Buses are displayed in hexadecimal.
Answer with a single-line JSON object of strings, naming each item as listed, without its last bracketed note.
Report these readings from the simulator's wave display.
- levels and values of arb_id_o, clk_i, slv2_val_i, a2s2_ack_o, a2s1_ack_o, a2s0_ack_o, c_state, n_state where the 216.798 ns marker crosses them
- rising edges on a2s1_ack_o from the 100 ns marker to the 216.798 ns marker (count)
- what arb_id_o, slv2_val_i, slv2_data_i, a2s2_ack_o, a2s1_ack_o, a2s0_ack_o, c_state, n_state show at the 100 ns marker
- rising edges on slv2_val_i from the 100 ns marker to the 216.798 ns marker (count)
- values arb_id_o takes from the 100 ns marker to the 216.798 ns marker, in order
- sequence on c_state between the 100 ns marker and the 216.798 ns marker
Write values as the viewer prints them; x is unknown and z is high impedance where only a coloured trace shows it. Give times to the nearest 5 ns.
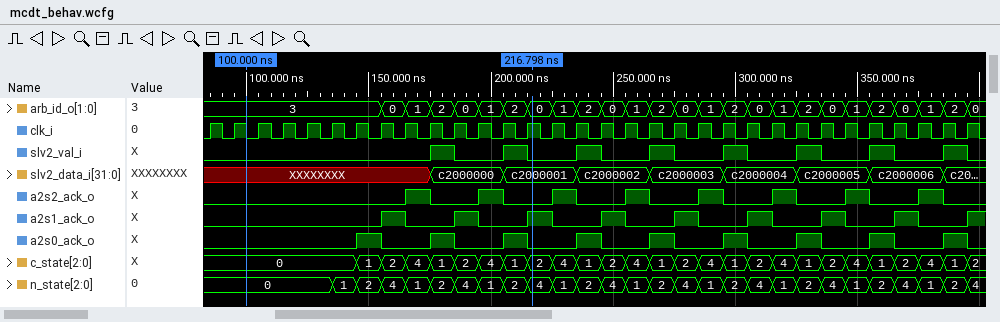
{"levels and values of arb_id_o, clk_i, slv2_val_i, a2s2_ack_o, a2s1_ack_o, a2s0_ack_o, c_state, n_state where the 216.798 ns marker crosses them": "arb_id_o=0, clk_i=1, slv2_val_i=0, a2s2_ack_o=0, a2s1_ack_o=1, a2s0_ack_o=0, c_state=2, n_state=4", "rising edges on a2s1_ack_o from the 100 ns marker to the 216.798 ns marker": "3", "what arb_id_o, slv2_val_i, slv2_data_i, a2s2_ack_o, a2s1_ack_o, a2s0_ack_o, c_state, n_state show at the 100 ns marker": "arb_id_o=3, slv2_val_i=0, slv2_data_i=XXXXXXXX, a2s2_ack_o=0, a2s1_ack_o=0, a2s0_ack_o=0, c_state=0, n_state=0", "rising edges on slv2_val_i from the 100 ns marker to the 216.798 ns marker": "2", "values arb_id_o takes from the 100 ns marker to the 216.798 ns marker, in order": "3, 0, 1, 2, 0, 1, 2, 0", "sequence on c_state between the 100 ns marker and the 216.798 ns marker": "0, 1, 2, 4, 1, 2, 4, 1, 2"}
